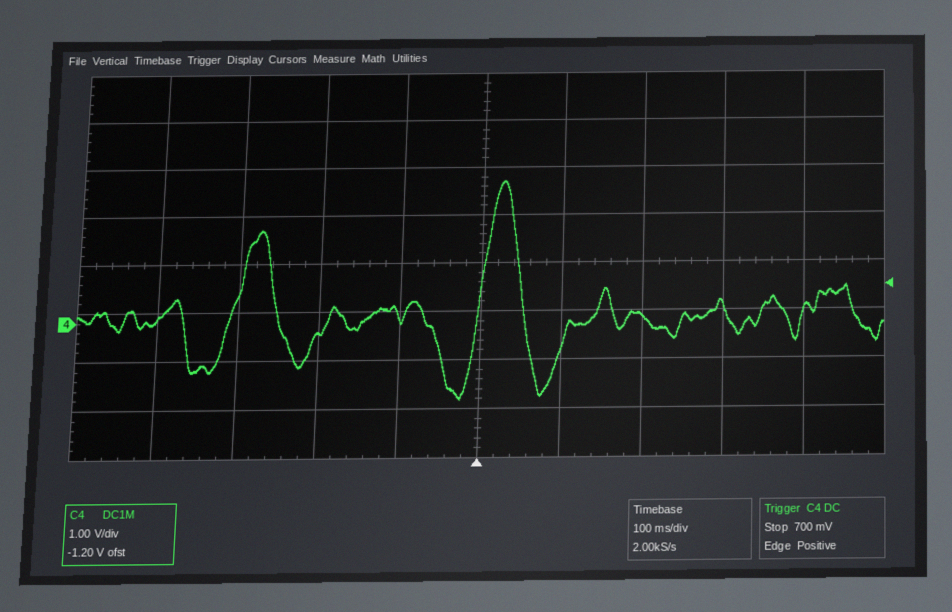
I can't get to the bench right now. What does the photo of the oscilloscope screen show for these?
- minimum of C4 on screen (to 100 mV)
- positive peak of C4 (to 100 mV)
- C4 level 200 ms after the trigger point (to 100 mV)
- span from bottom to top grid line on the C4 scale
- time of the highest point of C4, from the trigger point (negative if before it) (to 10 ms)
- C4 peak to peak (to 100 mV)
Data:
-1.6 V
2.9 V
100 mV
8 V
+30 ms
4.5 V
